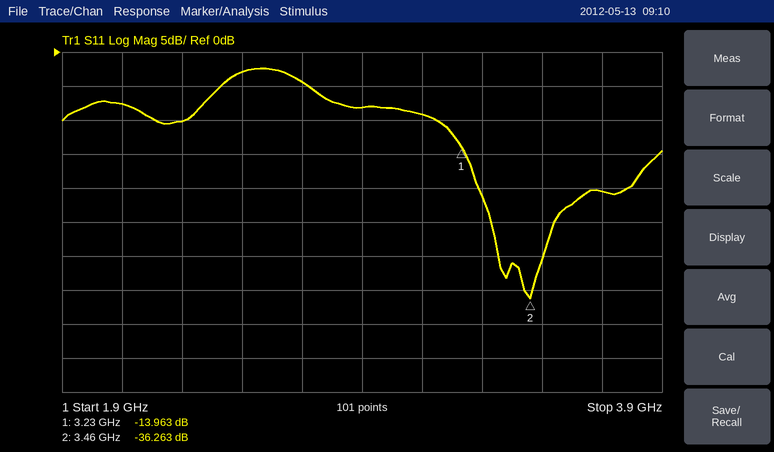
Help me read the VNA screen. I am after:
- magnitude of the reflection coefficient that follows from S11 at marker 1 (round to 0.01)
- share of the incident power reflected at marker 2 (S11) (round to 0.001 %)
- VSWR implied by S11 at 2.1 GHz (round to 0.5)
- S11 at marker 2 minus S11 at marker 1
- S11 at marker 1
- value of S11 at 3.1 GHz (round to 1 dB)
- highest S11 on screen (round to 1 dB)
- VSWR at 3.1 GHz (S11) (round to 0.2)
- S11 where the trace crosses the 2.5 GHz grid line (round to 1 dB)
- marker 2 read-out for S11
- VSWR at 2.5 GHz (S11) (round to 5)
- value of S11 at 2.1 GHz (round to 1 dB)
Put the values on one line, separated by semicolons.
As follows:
0.20; 0.024 %; 2.5; -22.300 dB; -13.963 dB; -9 dB; -2 dB; 2.0; -3 dB; -36.263 dB; 5; -8 dB
